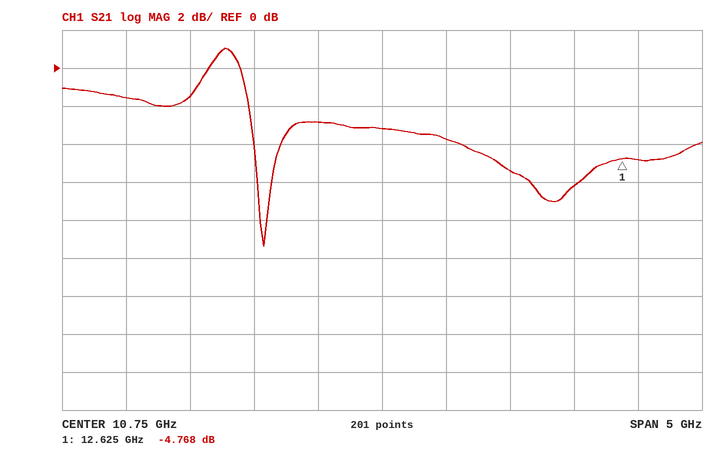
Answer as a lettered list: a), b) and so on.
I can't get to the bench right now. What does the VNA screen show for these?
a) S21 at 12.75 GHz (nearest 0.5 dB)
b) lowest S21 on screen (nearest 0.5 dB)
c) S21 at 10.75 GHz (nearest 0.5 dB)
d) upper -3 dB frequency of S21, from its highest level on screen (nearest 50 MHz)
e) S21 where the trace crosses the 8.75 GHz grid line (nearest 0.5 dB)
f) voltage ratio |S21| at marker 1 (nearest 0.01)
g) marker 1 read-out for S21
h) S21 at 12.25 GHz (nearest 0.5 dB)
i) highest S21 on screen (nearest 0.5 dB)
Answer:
a) -5.0 dB
b) -9.5 dB
c) -3.0 dB
d) 9.70 GHz
e) -1.5 dB
f) 0.58
g) -4.768 dB
h) -6.0 dB
i) 1.0 dB
